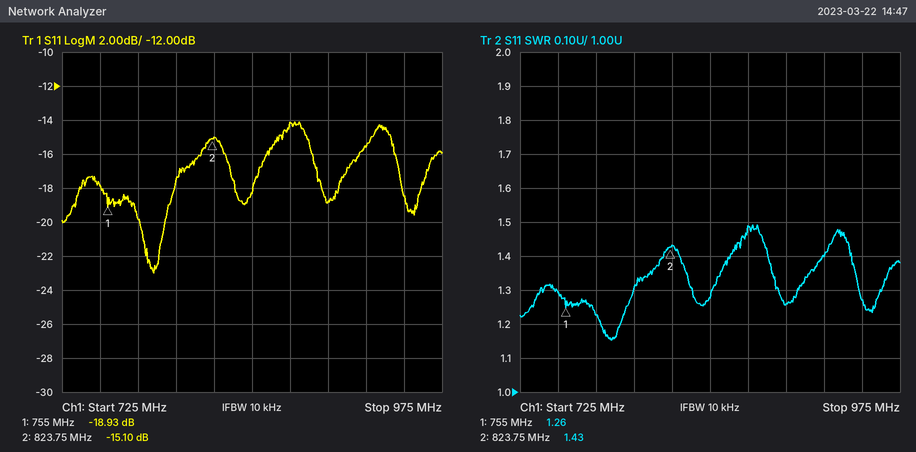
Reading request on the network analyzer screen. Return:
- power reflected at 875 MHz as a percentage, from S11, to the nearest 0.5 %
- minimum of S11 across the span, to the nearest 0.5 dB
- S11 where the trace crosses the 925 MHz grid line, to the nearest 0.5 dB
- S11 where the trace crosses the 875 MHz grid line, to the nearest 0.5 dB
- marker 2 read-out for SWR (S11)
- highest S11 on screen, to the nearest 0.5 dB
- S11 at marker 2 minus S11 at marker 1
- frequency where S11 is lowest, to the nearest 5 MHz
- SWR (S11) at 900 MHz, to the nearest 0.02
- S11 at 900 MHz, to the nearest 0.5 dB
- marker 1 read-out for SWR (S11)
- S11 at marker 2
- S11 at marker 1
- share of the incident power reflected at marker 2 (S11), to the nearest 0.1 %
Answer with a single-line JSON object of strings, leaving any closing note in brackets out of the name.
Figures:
{"power reflected at 875 MHz as a percentage, from S11, to the nearest 0.5 %": "4.0 %", "minimum of S11 across the span, to the nearest 0.5 dB": "-23.0 dB", "S11 where the trace crosses the 925 MHz grid line, to the nearest 0.5 dB": "-15.5 dB", "S11 where the trace crosses the 875 MHz grid line, to the nearest 0.5 dB": "-14.0 dB", "marker 2 read-out for SWR": "1.43", "highest S11 on screen, to the nearest 0.5 dB": "-14.0 dB", "S11 at marker 2 minus S11 at marker 1": "3.83 dB", "frequency where S11 is lowest, to the nearest 5 MHz": "785 MHz", "SWR (S11) at 900 MHz, to the nearest 0.02": "1.26", "S11 at 900 MHz, to the nearest 0.5 dB": "-19.0 dB", "marker 1 read-out for SWR": "1.26", "S11 at marker 2": "-15.10 dB", "S11 at marker 1": "-18.93 dB", "share of the incident power reflected at marker 2 (S11), to the nearest 0.1 %": "3.1 %"}
